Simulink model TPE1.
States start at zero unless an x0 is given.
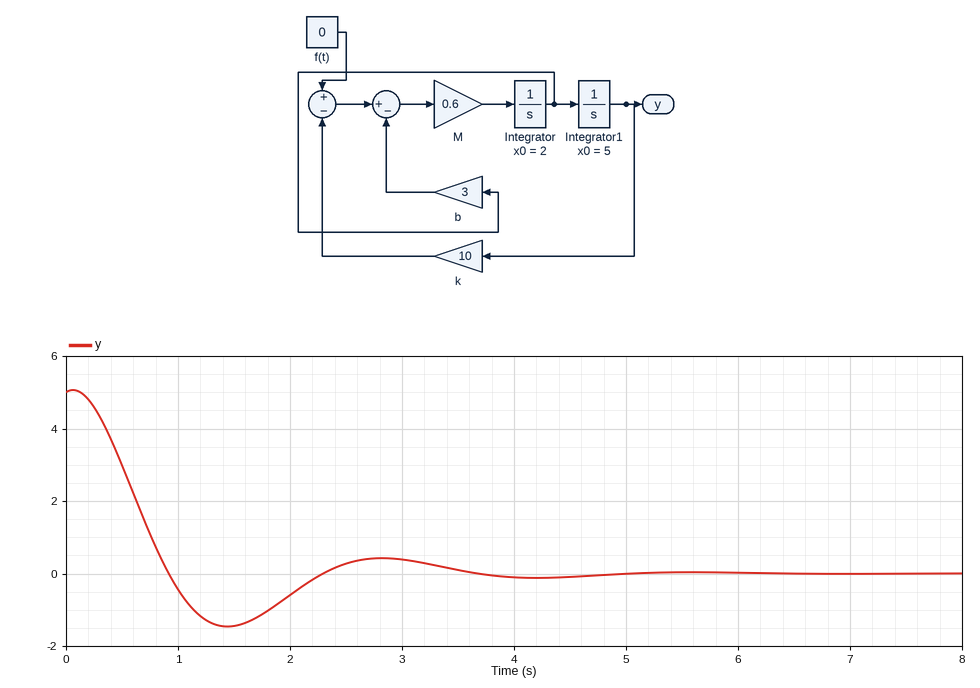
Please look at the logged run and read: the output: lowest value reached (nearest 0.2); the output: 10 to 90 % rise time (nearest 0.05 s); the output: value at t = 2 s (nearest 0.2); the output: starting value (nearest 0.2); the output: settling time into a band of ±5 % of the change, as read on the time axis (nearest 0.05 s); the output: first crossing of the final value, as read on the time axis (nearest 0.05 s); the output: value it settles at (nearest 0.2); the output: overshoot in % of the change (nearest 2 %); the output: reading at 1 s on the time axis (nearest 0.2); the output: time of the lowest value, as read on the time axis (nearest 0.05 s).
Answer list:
-1.4
0.55 s
-0.6
5.0
3.25 s
0.90 s
0.0
30 %
-0.4
1.45 s
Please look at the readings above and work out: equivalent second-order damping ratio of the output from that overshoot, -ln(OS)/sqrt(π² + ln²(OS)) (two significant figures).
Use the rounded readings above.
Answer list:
0.36
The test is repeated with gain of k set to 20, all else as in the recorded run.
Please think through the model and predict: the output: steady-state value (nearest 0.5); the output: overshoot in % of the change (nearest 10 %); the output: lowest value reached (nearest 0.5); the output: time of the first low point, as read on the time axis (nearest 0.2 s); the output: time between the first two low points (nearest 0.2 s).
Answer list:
0.0
40 %
-2.0
1.0 s
1.8 s
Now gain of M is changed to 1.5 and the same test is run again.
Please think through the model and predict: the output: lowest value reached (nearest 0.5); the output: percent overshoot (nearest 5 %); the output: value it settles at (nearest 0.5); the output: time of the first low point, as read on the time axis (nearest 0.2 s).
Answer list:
-0.5
10 %
0.0
1.0 s
